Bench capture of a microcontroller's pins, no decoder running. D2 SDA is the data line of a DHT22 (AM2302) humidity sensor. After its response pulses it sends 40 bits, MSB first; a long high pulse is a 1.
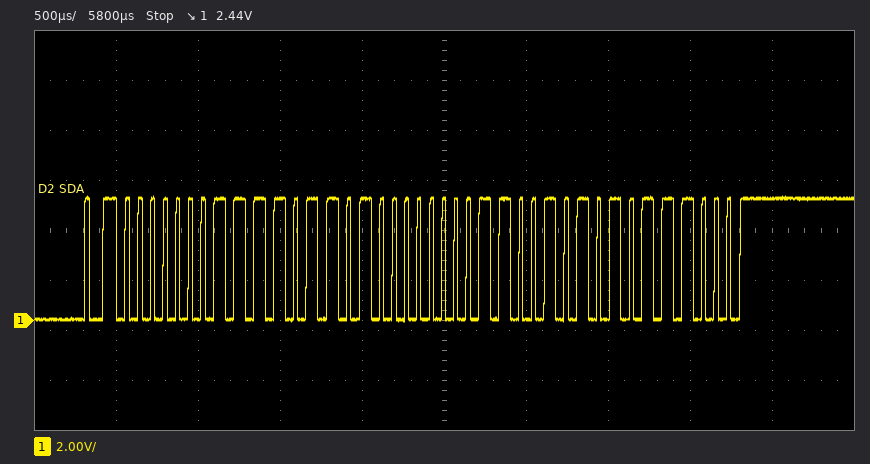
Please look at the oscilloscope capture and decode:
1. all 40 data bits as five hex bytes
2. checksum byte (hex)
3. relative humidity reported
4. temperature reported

01 ED 00 CA B8
0xB8
49.3 %
20.2 °C
